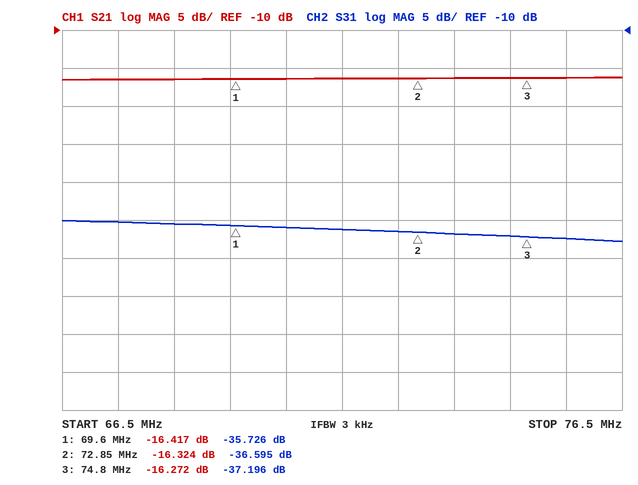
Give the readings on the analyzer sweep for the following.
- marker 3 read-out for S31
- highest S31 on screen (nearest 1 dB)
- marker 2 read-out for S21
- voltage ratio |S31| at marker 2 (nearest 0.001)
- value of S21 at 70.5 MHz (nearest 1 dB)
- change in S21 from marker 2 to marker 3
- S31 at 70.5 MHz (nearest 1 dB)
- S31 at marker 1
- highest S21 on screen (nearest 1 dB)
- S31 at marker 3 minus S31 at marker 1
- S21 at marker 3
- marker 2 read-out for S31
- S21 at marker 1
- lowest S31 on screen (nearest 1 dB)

-37.196 dB
-35 dB
-16.324 dB
0.015
-16 dB
0.052 dB
-36 dB
-35.726 dB
-16 dB
-1.470 dB
-16.272 dB
-36.595 dB
-16.417 dB
-38 dB
